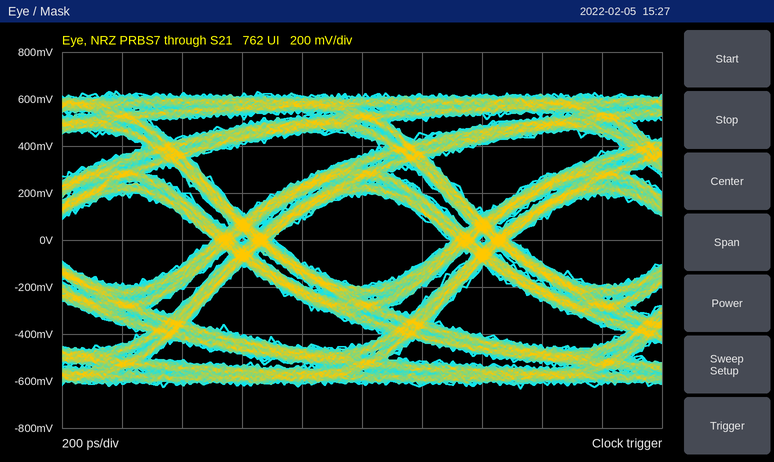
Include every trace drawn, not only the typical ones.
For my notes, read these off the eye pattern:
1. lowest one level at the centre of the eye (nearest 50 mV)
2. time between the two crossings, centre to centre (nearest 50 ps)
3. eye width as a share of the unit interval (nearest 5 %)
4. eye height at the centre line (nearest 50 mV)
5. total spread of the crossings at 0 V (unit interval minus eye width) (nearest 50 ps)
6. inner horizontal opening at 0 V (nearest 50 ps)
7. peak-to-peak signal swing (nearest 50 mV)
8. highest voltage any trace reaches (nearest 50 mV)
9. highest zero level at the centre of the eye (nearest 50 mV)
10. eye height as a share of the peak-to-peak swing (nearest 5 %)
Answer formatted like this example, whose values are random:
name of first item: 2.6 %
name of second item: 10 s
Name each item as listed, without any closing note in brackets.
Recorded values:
lowest one level at the centre of the eye: 200 mV
time between the two crossings, centre to centre: 800 ps
eye width as a share of the unit interval: 75 %
eye height at the centre line: 400 mV
total spread of the crossings at 0 V (unit interval minus eye width): 200 ps
inner horizontal opening at 0 V: 600 ps
peak-to-peak signal swing: 1.25 V
highest voltage any trace reaches: 650 mV
highest zero level at the centre of the eye: -200 mV
eye height as a share of the peak-to-peak swing: 30 %
